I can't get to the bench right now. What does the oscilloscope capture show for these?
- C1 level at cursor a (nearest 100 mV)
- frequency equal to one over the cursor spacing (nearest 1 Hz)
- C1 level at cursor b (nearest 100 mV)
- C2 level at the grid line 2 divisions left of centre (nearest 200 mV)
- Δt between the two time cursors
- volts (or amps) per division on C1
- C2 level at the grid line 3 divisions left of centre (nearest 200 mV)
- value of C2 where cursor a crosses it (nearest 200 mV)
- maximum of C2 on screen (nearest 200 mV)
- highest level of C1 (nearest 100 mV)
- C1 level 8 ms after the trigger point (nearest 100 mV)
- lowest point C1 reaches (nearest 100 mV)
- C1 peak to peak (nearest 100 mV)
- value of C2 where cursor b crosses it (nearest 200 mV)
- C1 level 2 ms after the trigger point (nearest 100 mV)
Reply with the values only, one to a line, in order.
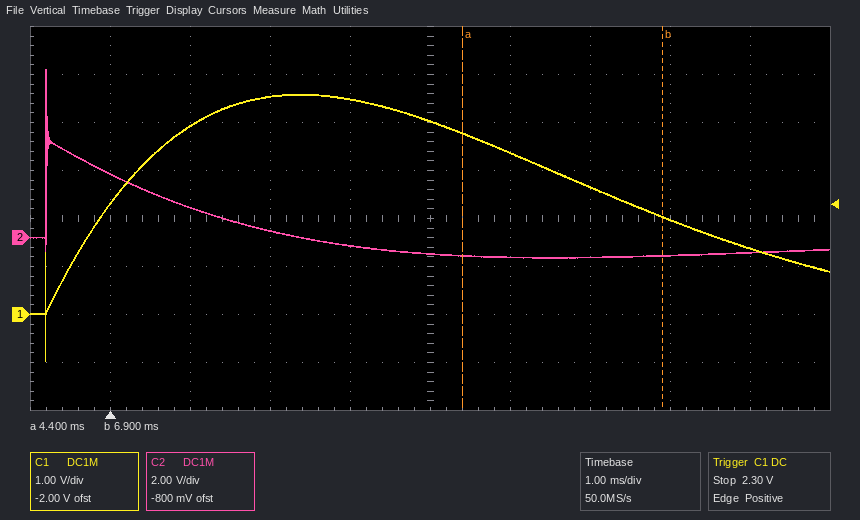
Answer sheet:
3.8 V
400 Hz
2.0 V
200 mV
2.5 ms
1 V
1.2 V
-800 mV
7.0 V
4.6 V
1.4 V
-1.0 V
5.6 V
-800 mV
4.5 V
